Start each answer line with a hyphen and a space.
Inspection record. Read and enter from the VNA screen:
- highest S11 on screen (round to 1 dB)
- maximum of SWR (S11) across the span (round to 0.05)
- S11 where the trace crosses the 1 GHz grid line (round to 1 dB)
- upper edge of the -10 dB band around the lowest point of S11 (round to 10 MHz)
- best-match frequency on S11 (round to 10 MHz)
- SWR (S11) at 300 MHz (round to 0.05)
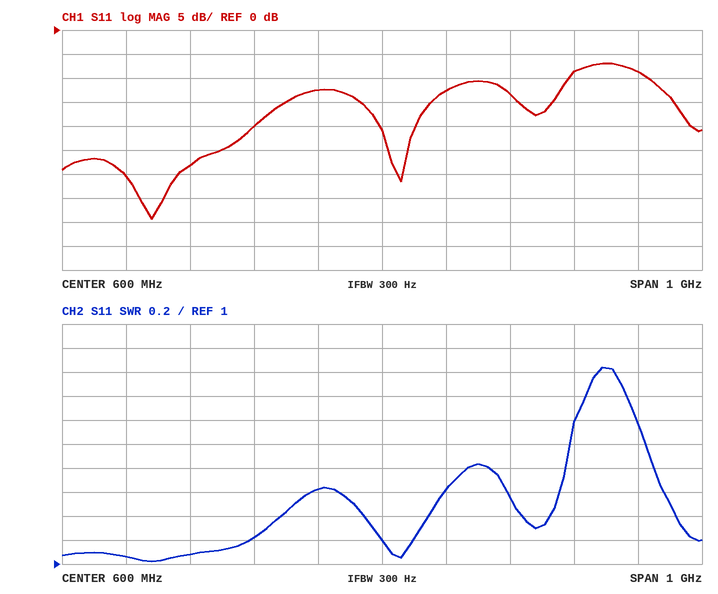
- -7 dB
- 2.65
- -9 dB
- 890 MHz
- 240 MHz
- 1.10
